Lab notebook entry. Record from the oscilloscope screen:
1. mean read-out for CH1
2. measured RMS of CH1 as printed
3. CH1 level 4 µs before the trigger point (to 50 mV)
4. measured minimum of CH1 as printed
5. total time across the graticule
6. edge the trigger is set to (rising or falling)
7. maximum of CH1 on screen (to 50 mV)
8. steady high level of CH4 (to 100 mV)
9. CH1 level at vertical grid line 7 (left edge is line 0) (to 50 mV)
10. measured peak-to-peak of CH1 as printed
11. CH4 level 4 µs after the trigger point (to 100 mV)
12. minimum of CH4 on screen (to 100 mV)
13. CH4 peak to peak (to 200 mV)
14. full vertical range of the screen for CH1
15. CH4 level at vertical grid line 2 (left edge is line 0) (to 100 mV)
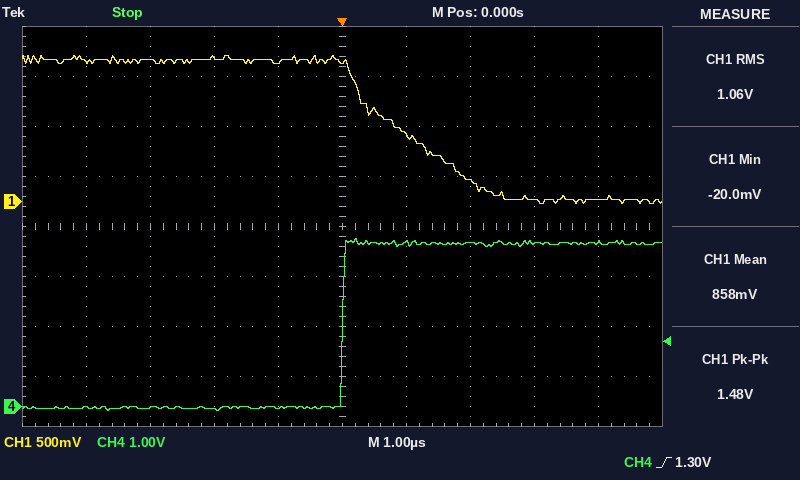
858 mV
1.06 V
1.40 V
-20.0 mV
10 µs
rising
1.45 V
3.3 V
200 mV
1.48 V
3.3 V
-100 mV
3.4 V
4 V
0.0 V
